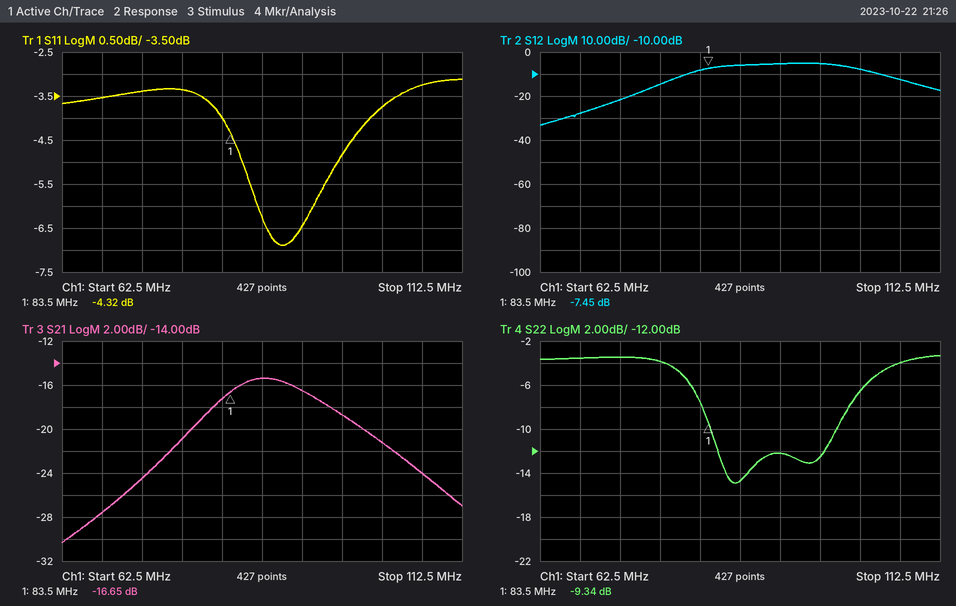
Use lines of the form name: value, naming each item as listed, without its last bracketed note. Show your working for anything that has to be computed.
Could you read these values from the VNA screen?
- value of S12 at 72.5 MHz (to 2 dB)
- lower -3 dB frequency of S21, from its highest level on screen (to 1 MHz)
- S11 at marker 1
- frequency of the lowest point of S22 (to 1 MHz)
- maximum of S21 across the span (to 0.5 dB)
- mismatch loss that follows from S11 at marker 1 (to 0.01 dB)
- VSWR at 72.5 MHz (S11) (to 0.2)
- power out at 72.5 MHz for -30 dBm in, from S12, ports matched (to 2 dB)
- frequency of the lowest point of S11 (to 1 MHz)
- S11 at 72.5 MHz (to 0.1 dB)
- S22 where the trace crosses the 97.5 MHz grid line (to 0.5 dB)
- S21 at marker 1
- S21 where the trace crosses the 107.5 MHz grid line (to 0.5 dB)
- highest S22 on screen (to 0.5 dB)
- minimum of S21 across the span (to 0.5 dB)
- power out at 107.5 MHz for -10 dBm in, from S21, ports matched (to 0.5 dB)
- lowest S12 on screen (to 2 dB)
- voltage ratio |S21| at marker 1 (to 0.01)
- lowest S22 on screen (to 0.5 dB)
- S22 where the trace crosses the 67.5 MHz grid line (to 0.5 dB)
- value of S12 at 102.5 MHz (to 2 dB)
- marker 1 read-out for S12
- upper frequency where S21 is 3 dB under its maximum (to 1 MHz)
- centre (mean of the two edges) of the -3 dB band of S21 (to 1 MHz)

value of S12 at 72.5 MHz: -22 dB
lower -3 dB frequency of S21, from its highest level on screen: 81 MHz
S11 at marker 1: -4.32 dB
frequency of the lowest point of S22: 87 MHz
maximum of S21 across the span: -15.5 dB
mismatch loss that follows from S11 at marker 1: −10 log10(1 − 10^(-4.32/10)) ≈ 2.01 dB
VSWR at 72.5 MHz (S11): |Γ| = 10^(-3.4/20) = 0.6761; VSWR = (1 + 0.6761)/(1 − 0.6761) ≈ 5.2
power out at 72.5 MHz for -30 dBm in, from S12, ports matched: -30 dBm + (-22 dB) = -52 dBm
frequency of the lowest point of S11: 90 MHz
S11 at 72.5 MHz: -3.4 dB
S22 where the trace crosses the 97.5 MHz grid line: -12.5 dB
S21 at marker 1: -16.65 dB
S21 where the trace crosses the 107.5 MHz grid line: -24.0 dB
highest S22 on screen: -3.5 dB
minimum of S21 across the span: -30.5 dB
power out at 107.5 MHz for -10 dBm in, from S21, ports matched: -10 dBm + (-24.0 dB) = -34.0 dBm
lowest S12 on screen: -34 dB
voltage ratio |S21| at marker 1: 10^(-16.65/20) ≈ 0.15
lowest S22 on screen: -15.0 dB
S22 where the trace crosses the 67.5 MHz grid line: -3.5 dB
value of S12 at 102.5 MHz: -8 dB
marker 1 read-out for S12: -7.45 dB
upper frequency where S21 is 3 dB under its maximum: 97 MHz
centre (mean of the two edges) of the -3 dB band of S21: 89 MHz
